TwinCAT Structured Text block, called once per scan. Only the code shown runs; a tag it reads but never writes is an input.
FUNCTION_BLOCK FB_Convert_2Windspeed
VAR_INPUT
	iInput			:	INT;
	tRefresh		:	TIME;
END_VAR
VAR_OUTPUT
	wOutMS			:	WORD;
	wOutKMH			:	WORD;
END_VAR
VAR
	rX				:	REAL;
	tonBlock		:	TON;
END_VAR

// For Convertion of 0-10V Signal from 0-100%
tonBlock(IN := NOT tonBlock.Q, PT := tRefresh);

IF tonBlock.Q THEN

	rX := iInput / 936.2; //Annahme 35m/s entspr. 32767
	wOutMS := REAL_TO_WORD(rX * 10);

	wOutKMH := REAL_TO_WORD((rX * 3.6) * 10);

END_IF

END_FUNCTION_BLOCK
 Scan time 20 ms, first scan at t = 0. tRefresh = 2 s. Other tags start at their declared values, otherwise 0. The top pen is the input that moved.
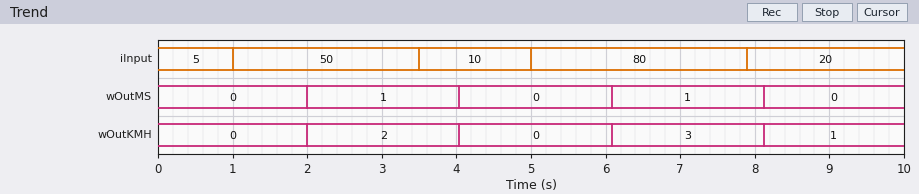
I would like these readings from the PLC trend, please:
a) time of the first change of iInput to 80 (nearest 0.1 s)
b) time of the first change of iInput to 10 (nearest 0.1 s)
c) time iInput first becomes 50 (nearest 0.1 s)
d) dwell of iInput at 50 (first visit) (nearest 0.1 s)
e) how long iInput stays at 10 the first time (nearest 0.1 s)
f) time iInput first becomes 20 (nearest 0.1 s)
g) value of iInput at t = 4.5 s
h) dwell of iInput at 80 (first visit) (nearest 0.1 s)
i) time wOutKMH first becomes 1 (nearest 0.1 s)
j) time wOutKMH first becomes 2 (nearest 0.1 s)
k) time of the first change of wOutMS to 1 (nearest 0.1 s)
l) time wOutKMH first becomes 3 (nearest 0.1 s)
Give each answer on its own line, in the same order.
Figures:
5.0 s
3.5 s
1.0 s
2.5 s
1.5 s
7.9 s
10
2.9 s
8.1 s
2.0 s
2.0 s
6.1 s
